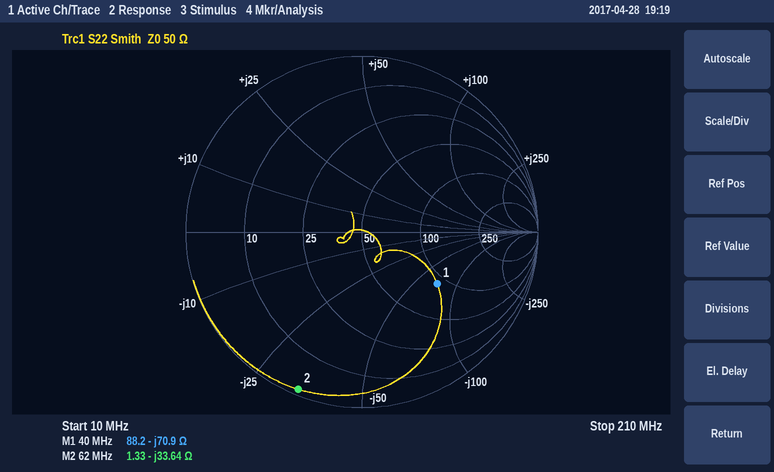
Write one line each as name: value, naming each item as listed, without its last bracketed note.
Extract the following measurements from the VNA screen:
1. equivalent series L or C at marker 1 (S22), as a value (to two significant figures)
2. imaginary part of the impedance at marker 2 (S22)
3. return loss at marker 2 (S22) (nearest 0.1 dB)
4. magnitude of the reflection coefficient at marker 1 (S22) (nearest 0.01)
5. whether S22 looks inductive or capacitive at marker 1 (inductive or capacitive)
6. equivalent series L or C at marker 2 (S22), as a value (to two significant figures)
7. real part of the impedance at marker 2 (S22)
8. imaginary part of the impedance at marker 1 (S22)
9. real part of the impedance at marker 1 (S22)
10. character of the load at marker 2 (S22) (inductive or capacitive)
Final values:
equivalent series L or C at marker 1 (S22), as a value: 56 pF
imaginary part of the impedance at marker 2: -33.64 Ω
return loss at marker 2 (S22): 0.3 dB
magnitude of the reflection coefficient at marker 1 (S22): 0.52
whether S22 looks inductive or capacitive at marker 1: capacitive
equivalent series L or C at marker 2 (S22), as a value: 76 pF
real part of the impedance at marker 2: 1.33 Ω
imaginary part of the impedance at marker 1: -70.9 Ω
real part of the impedance at marker 1: 88.2 Ω
character of the load at marker 2 (S22): capacitive
